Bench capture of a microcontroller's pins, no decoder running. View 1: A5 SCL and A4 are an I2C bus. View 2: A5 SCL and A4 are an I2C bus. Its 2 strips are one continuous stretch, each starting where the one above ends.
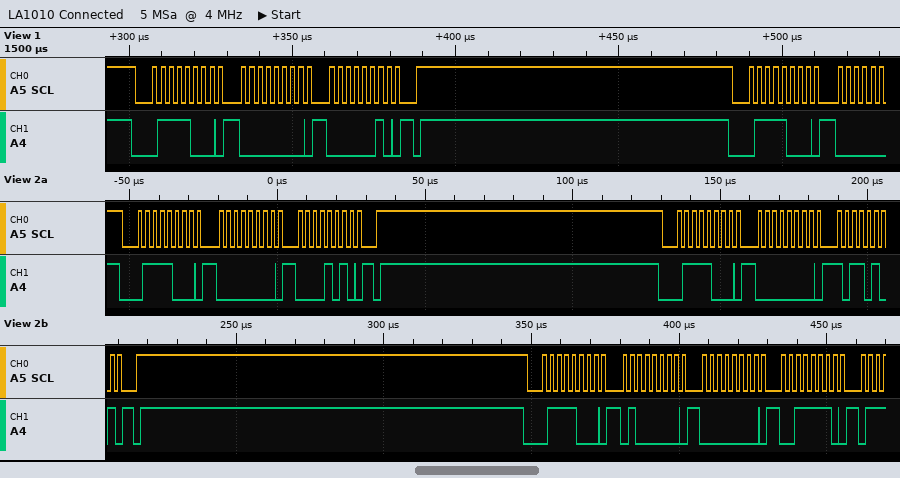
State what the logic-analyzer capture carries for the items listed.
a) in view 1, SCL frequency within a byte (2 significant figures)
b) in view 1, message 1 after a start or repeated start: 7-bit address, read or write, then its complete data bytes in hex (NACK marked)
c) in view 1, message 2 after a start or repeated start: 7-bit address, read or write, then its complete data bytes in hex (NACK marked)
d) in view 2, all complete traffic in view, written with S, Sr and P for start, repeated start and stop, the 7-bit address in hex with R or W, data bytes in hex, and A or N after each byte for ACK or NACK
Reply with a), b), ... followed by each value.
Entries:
a) 400 kHz
b) 0x3C write: 00 02
c) 0x3C write
d) S 3CW A 00 A 0A A P S 3CW A 00 A B5 A P S 3CW A 40 A 00 A 3E A
